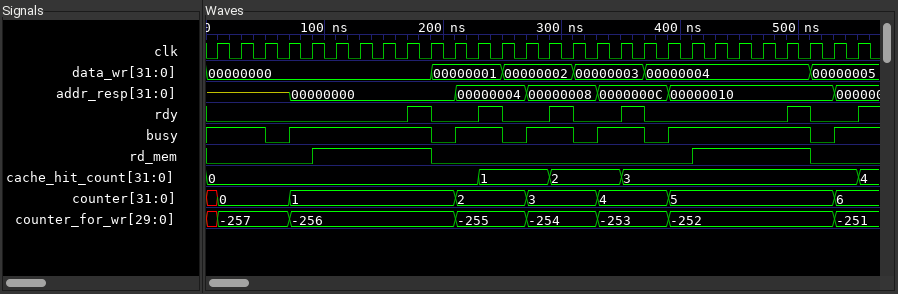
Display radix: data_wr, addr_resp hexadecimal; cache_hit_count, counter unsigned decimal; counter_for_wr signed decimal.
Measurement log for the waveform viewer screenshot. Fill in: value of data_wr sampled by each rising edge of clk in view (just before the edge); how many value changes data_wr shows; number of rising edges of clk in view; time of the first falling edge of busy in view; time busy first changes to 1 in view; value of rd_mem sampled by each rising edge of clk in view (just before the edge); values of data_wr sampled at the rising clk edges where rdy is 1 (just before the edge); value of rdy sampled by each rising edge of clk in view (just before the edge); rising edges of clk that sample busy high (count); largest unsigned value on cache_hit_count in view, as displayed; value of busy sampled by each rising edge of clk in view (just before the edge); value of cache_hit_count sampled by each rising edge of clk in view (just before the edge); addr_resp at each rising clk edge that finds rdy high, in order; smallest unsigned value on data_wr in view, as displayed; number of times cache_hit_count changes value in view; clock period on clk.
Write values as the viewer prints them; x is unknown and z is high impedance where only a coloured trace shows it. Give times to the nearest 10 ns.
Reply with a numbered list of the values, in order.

1. 00000000, 00000000, 00000000, 00000000, 00000000, 00000000, 00000000, 00000000, 00000000, 00000000, 00000001, 00000001, 00000001, 00000002, 00000002, 00000002, 00000003, 00000003, 00000003, 00000004, 00000004, 00000004, 00000004, 00000004, 00000004, 00000004, 00000005, 00000005
2. 5
3. 28
4. 50 ns
5. 70 ns
6. 0 0 0 0 0 1 1 1 1 1 0 0 0 0 0 0 0 0 0 0 0 1 1 1 1 1 0 0
7. 00000000, 00000001, 00000002, 00000003, 00000004
8. 0 0 0 0 0 0 0 0 0 1 0 0 1 0 0 1 0 0 1 0 0 0 0 0 0 1 0 0
9. 22
10. 4
11. 1 1 1 0 1 1 1 1 1 1 0 1 1 0 1 1 0 1 1 0 1 1 1 1 1 1 0 1
12. 0, 0, 0, 0, 0, 0, 0, 0, 0, 0, 0, 0, 1, 1, 1, 2, 2, 2, 3, 3, 3, 3, 3, 3, 3, 3, 3, 3
13. 00000000, 00000004, 00000008, 0000000C, 00000010
14. 00000000
15. 4
16. 20 ns
